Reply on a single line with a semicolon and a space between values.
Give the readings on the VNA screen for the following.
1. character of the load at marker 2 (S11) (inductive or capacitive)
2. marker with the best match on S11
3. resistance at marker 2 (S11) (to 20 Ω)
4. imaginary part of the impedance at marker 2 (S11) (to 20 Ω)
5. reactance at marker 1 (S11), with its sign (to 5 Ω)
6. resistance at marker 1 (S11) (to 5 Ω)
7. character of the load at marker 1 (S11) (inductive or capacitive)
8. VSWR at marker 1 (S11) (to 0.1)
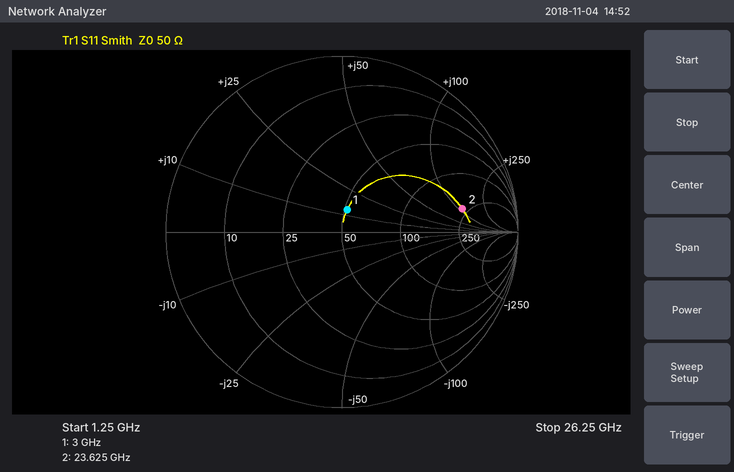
inductive; marker 1; 220 Ω; +120 Ω; +15 Ω; 50 Ω; inductive; 1.3
